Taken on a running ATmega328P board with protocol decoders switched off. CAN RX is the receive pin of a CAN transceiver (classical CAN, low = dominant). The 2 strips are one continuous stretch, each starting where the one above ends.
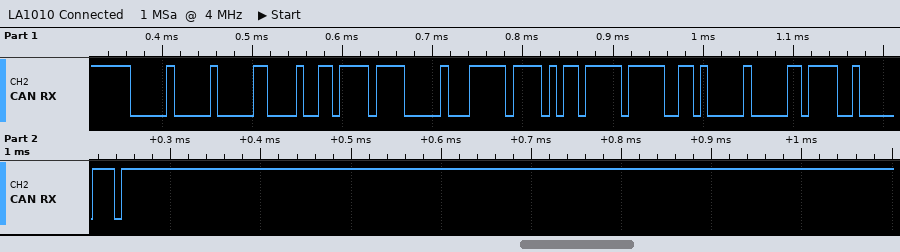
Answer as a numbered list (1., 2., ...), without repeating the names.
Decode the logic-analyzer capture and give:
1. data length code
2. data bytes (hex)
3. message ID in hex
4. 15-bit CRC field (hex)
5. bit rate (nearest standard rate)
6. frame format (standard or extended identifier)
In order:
1. 8
2. 4D EF 00 FF AD FF B4 00
3. 0x000
4. 0x5E41
5. 125 kbit/s
6. standard
